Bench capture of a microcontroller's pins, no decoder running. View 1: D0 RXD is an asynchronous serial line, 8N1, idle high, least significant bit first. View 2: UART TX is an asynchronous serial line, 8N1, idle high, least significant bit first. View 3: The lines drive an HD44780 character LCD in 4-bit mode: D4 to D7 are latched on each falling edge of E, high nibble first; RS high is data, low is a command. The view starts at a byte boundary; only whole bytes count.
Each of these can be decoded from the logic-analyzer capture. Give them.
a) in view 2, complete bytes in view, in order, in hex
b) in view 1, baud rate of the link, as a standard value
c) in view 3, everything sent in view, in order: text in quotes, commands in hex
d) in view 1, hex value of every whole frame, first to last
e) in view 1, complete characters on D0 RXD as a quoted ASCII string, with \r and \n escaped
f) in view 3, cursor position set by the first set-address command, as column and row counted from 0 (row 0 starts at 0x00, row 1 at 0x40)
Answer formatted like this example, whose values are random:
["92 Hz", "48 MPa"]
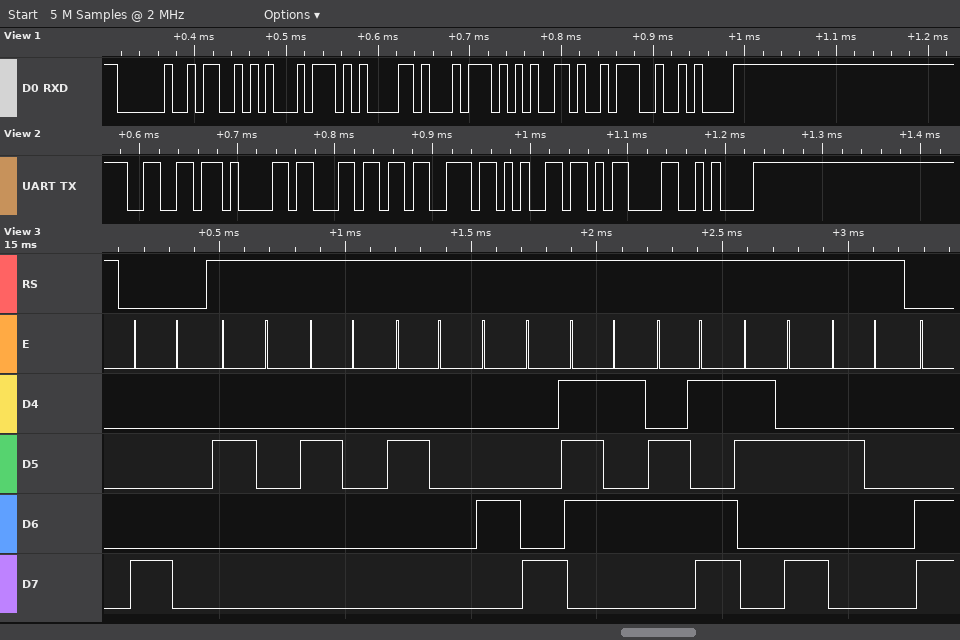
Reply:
["66 61 6C 73 65 0D 0A", "115200 baud", "0x80 \"   Hum: \"", "0x20 0x53 0x74 0x61 0x74 0x65 0x3A 0x0A", "\" State:\\n\"", "column 0, row 0"]
